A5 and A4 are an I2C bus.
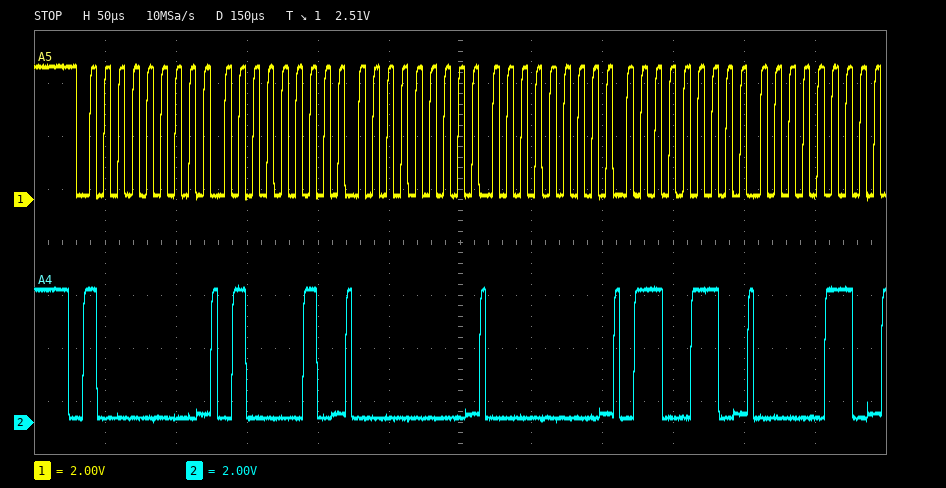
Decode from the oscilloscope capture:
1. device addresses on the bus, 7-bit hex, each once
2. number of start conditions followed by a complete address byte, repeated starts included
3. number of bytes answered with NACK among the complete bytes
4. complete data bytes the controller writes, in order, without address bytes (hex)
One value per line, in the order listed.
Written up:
0x40
1
0
42 00 00 66 06
